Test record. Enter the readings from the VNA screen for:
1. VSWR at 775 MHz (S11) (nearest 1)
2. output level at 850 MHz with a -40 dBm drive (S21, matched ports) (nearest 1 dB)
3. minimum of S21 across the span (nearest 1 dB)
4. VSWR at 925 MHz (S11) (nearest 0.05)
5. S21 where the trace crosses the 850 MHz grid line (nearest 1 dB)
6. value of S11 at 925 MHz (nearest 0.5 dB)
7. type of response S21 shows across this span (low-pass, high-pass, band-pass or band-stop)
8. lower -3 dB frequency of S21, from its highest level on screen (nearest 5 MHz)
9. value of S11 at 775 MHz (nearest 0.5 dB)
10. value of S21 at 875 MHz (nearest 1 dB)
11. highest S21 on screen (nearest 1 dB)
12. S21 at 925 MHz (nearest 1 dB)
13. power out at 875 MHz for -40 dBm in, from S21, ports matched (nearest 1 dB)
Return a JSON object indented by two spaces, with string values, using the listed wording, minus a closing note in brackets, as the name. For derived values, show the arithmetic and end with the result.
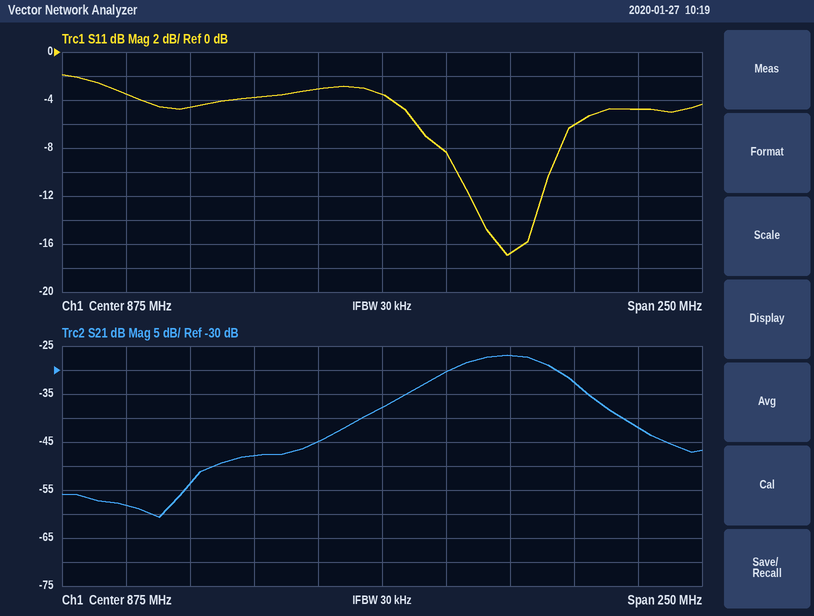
{
  "VSWR at 775 MHz (S11)": "|Γ| = 10^(-3.5/20) = 0.6683; VSWR = (1 + 0.6683)/(1 − 0.6683) ≈ 5",
  "output level at 850 MHz with a -40 dBm drive (S21, matched ports)": "-40 dBm + (-45 dB) = -85 dBm",
  "minimum of S21 across the span": "-61 dB",
  "VSWR at 925 MHz (S11)": "|Γ| = 10^(-17/20) = 0.1413; VSWR = (1 + 0.1413)/(1 − 0.1413) ≈ 1.33, so 1.35 to the nearest 0.05",
  "S21 where the trace crosses the 850 MHz grid line": "-45 dB",
  "value of S11 at 925 MHz": "-17.0 dB",
  "type of response S21 shows across this span": "band-pass",
  "lower -3 dB frequency of S21, from its highest level on screen": "900 MHz",
  "value of S11 at 775 MHz": "-3.5 dB",
  "value of S21 at 875 MHz": "-38 dB",
  "highest S21 on screen": "-27 dB",
  "S21 at 925 MHz": "-27 dB",
  "power out at 875 MHz for -40 dBm in, from S21, ports matched": "-40 dBm + (-38 dB) = -78 dBm"
}
